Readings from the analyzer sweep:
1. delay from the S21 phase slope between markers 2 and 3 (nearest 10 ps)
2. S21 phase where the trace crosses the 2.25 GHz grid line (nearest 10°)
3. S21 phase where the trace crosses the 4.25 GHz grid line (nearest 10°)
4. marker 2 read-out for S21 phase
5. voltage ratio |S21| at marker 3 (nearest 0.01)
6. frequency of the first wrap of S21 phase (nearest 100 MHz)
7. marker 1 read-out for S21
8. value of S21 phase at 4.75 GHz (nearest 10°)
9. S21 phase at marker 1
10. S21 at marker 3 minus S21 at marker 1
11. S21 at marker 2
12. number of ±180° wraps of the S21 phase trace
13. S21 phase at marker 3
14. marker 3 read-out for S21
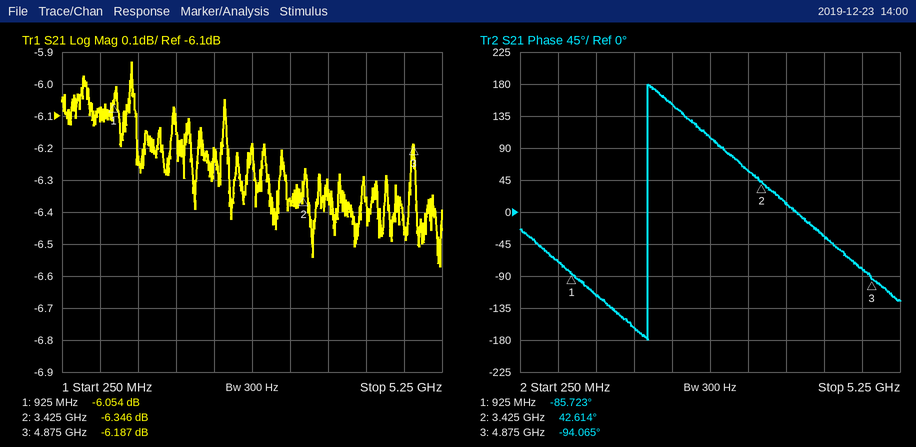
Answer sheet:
260 ps
150°
-30°
42.614°
0.49
1.9 GHz
-6.054 dB
-80°
-85.723°
-0.133 dB
-6.346 dB
1
-94.065°
-6.187 dB
